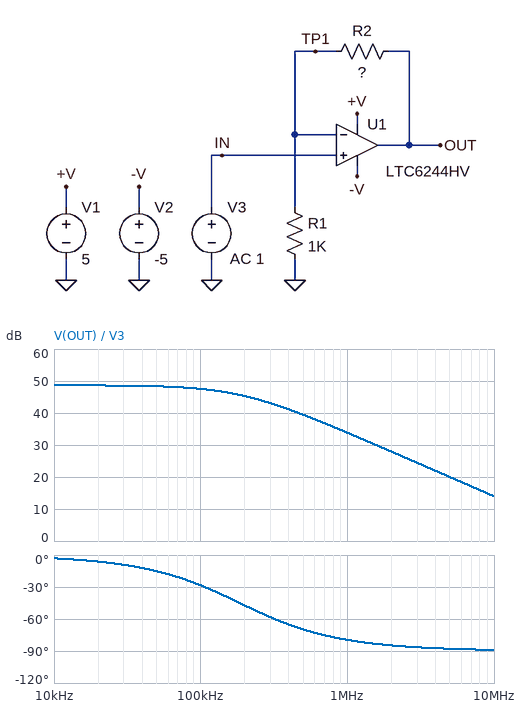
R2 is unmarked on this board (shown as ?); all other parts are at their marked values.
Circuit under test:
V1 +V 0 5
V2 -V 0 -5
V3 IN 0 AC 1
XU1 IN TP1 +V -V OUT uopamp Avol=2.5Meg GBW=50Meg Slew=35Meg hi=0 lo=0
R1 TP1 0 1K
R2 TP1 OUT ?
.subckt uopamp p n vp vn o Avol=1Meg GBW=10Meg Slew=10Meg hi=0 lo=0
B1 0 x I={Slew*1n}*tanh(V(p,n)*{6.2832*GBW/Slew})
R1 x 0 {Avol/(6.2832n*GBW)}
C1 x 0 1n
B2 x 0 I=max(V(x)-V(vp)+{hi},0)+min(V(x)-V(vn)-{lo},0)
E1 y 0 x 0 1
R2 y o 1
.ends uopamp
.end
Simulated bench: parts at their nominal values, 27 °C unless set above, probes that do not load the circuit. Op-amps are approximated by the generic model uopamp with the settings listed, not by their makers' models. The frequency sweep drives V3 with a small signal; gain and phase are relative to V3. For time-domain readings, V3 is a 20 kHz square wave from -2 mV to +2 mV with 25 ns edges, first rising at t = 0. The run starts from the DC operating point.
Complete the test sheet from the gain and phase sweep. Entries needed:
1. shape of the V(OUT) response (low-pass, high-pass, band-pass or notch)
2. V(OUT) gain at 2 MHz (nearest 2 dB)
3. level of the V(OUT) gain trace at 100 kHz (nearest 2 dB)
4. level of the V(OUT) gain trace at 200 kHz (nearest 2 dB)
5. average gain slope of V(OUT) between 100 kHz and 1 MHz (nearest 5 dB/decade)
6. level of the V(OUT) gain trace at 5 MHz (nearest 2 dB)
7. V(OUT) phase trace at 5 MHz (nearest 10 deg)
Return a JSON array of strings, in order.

["low-pass", "28 dB", "48 dB", "46 dB", "-15 dB/decade", "20 dB", "-90 deg"]
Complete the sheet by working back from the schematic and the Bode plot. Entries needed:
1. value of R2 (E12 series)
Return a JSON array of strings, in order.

["270 kΩ"]
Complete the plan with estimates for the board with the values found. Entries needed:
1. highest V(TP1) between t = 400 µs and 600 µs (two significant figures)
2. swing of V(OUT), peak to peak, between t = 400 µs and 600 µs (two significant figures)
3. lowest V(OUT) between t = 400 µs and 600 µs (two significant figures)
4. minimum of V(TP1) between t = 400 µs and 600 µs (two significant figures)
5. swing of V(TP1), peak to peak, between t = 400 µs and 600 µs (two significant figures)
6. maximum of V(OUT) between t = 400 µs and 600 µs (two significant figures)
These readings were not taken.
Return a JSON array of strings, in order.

["2.0 mV", "1.1 V", "-540 mV", "-2.0 mV", "4.0 mV", "540 mV"]
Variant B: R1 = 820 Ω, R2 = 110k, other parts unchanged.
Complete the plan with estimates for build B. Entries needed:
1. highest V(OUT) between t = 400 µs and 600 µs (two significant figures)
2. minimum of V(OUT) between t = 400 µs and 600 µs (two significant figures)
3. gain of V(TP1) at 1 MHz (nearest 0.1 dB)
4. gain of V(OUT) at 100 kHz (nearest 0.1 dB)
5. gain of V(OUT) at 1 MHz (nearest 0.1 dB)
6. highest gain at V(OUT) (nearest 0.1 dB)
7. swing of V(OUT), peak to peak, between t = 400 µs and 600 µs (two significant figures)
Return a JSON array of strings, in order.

["270 mV", "-270 mV", "-9.2 dB", "42.3 dB", "33.4 dB", "42.6 dB", "540 mV"]
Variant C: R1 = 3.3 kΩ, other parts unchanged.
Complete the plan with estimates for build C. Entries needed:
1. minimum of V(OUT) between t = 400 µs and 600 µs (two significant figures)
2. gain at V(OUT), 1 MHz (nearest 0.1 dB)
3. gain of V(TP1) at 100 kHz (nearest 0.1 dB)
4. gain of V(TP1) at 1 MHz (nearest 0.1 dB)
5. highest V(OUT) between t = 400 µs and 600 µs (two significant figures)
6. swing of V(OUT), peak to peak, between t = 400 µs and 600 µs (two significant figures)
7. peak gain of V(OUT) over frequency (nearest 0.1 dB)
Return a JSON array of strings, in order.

["-170 mV", "32.6 dB", "-0.1 dB", "-5.7 dB", "170 mV", "330 mV", "38.4 dB"]
